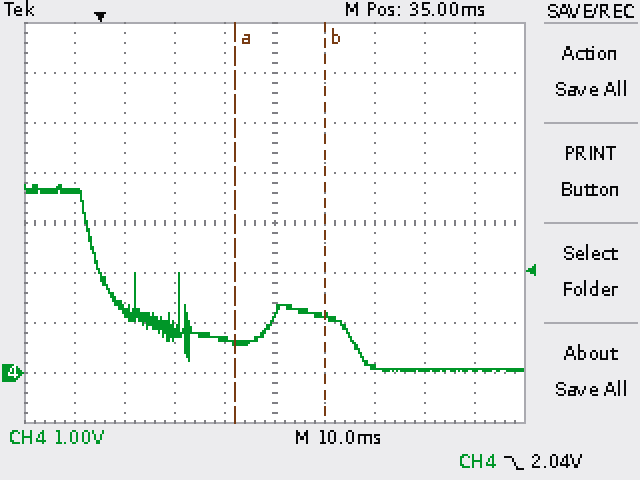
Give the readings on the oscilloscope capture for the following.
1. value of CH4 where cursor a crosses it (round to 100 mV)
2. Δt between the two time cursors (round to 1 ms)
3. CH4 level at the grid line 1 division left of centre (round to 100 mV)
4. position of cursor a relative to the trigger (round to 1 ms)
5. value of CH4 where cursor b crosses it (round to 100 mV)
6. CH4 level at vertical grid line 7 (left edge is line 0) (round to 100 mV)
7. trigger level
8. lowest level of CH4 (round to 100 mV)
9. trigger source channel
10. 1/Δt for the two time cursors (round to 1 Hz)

600 mV
18 ms
700 mV
+27 ms
1.1 V
100 mV
2.04 V
0.0 V
CH4
56 Hz
